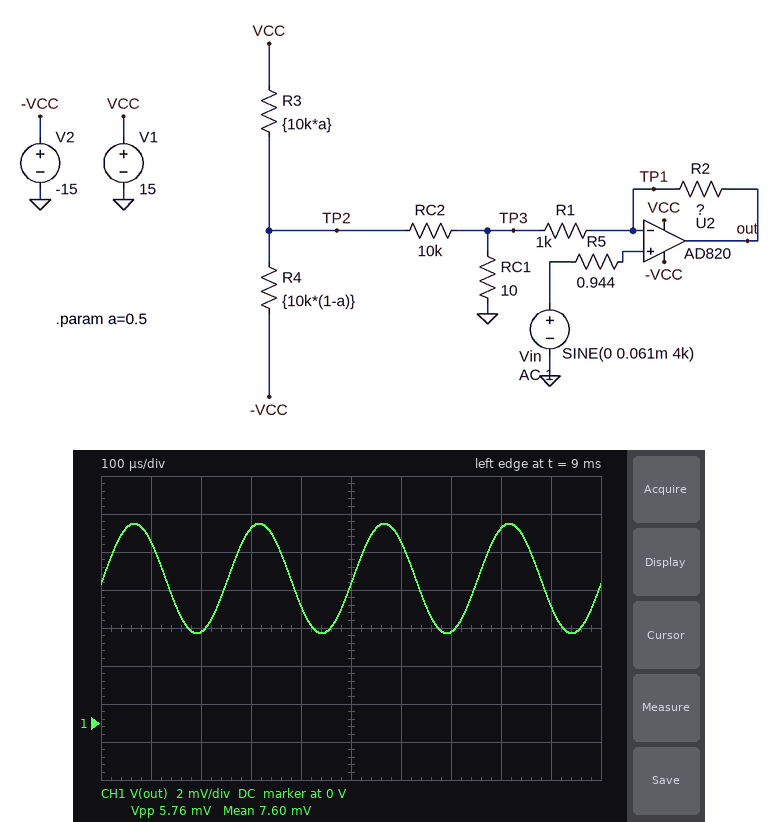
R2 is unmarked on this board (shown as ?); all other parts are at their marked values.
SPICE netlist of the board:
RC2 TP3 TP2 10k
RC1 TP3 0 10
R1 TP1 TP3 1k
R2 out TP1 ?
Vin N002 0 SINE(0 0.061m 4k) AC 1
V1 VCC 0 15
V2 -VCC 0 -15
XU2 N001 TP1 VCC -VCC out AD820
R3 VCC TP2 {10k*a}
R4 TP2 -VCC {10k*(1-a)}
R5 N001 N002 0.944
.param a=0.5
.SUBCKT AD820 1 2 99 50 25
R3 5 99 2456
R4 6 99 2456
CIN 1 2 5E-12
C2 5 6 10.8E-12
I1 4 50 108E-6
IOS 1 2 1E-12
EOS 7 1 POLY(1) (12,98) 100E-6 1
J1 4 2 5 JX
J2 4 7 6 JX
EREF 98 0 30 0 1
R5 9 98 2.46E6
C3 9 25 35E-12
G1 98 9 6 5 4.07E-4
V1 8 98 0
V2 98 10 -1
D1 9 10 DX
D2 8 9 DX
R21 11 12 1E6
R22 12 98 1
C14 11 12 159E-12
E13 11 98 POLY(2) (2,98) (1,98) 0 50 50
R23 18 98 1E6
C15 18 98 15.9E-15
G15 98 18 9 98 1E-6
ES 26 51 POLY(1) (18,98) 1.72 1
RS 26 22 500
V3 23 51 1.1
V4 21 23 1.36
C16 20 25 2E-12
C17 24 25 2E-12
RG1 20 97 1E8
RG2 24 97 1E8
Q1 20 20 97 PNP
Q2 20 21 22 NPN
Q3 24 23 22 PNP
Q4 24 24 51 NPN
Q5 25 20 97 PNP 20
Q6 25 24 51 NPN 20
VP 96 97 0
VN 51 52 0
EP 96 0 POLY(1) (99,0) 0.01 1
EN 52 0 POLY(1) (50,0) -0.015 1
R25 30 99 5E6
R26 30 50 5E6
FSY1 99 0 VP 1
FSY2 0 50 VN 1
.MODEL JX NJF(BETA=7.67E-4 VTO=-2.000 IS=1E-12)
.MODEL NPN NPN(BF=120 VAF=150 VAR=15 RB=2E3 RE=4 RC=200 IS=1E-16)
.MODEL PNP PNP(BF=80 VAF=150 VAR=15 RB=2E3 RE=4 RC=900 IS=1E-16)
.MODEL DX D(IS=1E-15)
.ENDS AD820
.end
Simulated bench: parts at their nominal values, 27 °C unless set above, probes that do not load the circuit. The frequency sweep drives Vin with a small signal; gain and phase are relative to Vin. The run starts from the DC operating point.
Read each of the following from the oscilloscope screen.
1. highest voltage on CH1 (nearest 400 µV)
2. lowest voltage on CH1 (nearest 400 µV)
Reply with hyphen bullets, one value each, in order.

- 10.4 mV
- 4.8 mV
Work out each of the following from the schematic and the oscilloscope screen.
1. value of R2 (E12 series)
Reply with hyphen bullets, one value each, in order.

- 47 kΩ
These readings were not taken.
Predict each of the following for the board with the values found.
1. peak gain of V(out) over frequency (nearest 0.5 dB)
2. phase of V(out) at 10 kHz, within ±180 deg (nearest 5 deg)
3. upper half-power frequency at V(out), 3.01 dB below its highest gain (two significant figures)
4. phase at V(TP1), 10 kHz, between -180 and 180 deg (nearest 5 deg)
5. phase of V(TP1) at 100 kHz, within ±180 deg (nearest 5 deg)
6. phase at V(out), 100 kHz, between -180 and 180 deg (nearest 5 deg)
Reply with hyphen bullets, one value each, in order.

- 33.5 dB
- -15 deg
- 40 kHz
- -15 deg
- -70 deg
- -70 deg
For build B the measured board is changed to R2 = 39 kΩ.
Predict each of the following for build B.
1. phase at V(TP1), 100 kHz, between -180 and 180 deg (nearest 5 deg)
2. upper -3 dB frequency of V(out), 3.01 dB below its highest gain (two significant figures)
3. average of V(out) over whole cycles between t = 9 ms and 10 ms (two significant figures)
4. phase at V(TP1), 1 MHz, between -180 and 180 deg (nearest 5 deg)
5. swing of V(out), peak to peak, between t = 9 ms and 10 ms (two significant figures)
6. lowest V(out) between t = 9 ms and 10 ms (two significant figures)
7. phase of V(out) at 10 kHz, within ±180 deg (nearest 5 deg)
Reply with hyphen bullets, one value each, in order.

- -65 deg
- 48 kHz
- 6.3 mV
- -140 deg
- 4.8 mV
- 3.9 mV
- -10 deg
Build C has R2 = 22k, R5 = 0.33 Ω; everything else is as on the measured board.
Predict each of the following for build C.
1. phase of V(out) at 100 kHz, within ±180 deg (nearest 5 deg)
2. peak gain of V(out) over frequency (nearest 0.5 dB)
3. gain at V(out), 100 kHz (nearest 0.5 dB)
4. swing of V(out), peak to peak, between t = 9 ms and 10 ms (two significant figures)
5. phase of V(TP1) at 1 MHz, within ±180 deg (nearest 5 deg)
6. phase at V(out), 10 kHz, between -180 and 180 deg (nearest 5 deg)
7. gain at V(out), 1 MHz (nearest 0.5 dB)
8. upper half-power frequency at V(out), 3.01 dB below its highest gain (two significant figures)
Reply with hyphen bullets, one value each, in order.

- -50 deg
- 27.0 dB
- 23.5 dB
- 2.8 mV
- -115 deg
- -5 deg
- 5.0 dB
- 84 kHz
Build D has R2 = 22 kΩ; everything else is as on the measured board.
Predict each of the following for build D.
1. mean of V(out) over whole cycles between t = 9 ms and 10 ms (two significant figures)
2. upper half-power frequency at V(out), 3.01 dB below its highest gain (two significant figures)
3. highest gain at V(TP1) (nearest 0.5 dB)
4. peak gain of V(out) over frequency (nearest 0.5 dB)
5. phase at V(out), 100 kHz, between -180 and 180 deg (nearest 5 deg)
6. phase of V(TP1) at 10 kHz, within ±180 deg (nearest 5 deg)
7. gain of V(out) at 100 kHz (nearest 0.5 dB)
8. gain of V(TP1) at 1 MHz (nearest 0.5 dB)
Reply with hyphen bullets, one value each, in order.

- 3.6 mV
- 84 kHz
- 0 dB
- 27.0 dB
- -50 deg
- -5 deg
- 23.5 dB
- -26.0 dB
